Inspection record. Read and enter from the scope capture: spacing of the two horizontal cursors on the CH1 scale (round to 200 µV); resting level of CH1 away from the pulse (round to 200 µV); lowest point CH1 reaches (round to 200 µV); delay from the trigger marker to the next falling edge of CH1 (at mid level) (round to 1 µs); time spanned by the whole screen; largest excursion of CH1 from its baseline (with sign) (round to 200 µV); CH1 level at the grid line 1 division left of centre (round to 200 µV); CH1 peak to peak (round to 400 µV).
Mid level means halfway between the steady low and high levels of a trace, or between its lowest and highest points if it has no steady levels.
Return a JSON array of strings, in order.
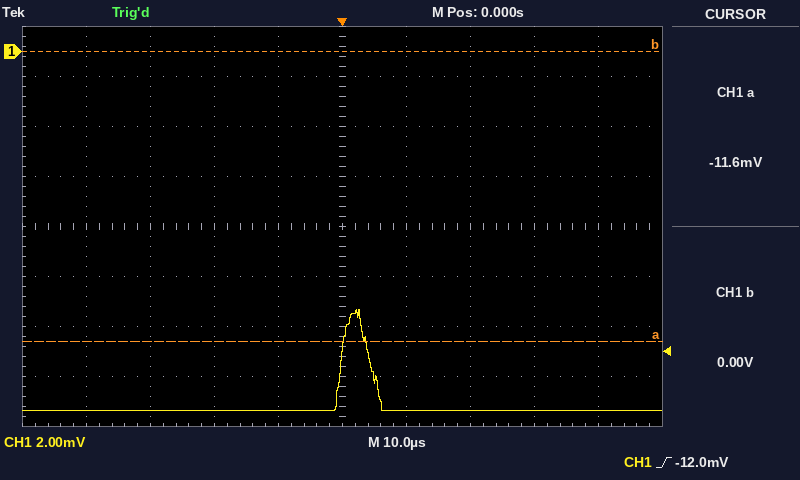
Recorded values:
["11.6 mV", "-14.4 mV", "-14.4 mV", "4 µs", "100 µs", "+4.0 mV", "-14.4 mV", "4.0 mV"]
